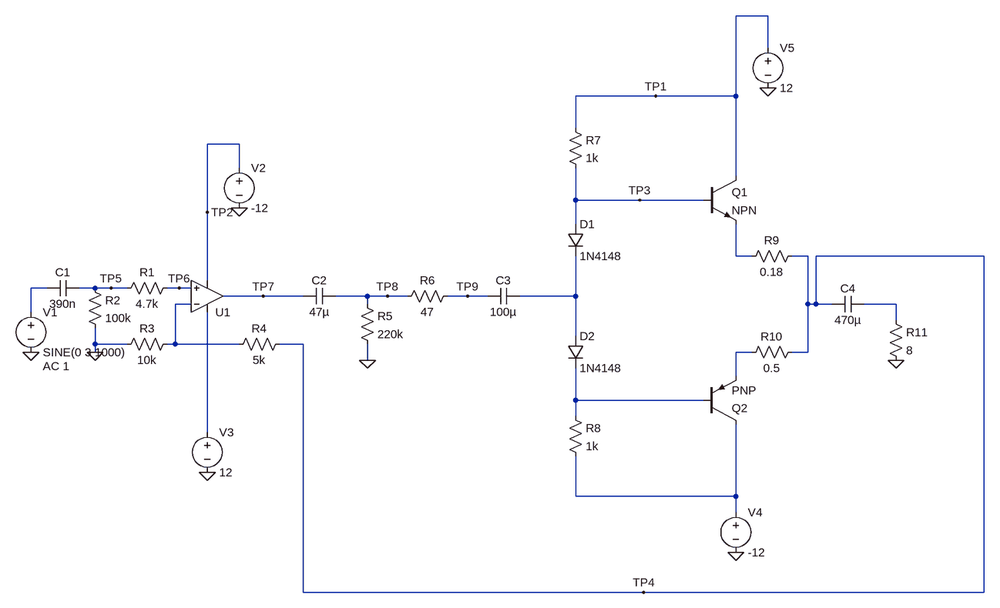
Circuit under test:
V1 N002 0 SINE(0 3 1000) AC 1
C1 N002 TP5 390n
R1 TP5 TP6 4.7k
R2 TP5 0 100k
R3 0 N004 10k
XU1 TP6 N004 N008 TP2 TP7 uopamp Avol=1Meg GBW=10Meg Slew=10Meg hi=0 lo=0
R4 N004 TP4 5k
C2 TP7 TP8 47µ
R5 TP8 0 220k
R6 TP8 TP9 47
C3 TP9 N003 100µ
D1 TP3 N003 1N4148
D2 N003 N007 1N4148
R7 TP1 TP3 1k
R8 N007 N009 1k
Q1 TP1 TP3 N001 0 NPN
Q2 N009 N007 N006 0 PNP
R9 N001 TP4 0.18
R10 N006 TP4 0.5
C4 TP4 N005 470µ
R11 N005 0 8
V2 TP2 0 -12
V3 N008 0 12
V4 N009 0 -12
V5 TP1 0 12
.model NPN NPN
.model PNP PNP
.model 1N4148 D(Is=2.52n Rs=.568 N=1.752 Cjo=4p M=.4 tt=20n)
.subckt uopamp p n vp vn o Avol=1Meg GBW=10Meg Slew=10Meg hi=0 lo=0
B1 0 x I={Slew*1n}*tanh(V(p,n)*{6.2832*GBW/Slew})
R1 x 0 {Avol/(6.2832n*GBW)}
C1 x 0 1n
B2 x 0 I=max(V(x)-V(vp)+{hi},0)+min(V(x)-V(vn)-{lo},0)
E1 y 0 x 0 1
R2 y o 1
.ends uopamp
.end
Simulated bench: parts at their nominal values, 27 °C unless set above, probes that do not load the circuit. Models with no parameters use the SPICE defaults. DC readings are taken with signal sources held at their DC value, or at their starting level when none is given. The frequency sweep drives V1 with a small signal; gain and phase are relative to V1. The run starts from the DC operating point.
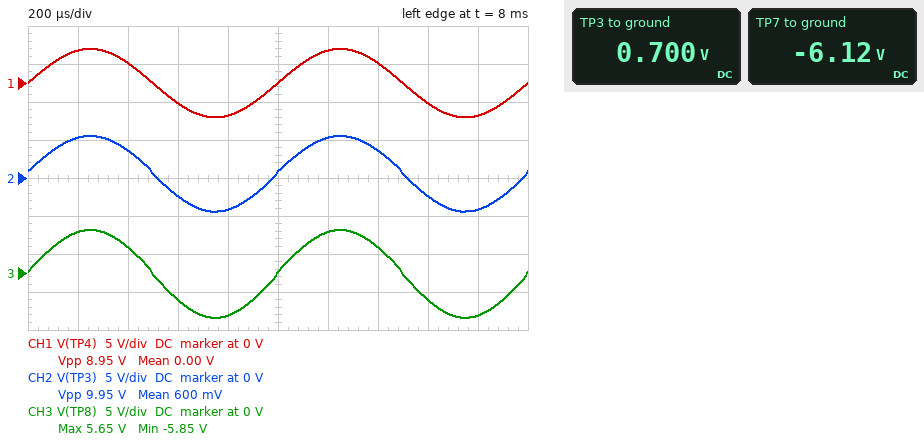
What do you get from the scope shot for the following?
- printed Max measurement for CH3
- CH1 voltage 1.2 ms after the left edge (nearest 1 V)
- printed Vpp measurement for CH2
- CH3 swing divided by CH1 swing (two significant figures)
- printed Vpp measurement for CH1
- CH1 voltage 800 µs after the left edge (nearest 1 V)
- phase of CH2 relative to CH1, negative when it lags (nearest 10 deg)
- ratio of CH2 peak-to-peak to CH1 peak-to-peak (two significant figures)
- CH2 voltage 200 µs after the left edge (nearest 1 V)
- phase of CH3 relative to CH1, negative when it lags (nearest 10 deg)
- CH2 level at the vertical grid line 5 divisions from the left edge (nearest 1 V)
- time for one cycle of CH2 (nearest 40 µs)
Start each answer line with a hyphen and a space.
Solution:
- 5.65 V
- 4 V
- 9.95 V
- 1.3
- 8.95 V
- -4 V
- 0 deg
- 1.1
- 5 V
- 0 deg
- 1 V
- 1.00 ms
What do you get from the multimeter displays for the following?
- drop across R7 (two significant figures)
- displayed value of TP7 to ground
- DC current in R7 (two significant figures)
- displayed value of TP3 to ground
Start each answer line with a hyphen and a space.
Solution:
- 11 V
- -6.12 V
- 11 mA
- 0.700 V
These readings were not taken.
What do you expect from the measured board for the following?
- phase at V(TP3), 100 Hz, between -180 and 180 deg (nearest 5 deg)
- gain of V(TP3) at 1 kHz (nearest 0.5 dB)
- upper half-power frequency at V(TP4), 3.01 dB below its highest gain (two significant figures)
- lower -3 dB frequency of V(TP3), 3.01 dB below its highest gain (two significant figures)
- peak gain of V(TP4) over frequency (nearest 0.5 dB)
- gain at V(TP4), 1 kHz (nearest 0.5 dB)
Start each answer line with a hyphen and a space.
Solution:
- 25 deg
- 32.5 dB
- 210 kHz
- 43 Hz
- 3.5 dB
- 3.5 dB
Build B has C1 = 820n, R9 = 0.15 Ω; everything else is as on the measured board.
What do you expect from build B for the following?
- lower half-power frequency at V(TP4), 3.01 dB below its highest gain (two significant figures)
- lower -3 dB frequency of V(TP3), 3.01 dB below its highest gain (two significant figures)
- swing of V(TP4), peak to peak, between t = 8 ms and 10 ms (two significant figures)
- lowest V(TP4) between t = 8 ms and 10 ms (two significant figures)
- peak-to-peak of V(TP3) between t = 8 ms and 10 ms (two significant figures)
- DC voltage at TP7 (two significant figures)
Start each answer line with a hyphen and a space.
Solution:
- 1.9 Hz
- 42 Hz
- 8.6 V
- -4.1 V
- 9.5 V
- -6.7 V
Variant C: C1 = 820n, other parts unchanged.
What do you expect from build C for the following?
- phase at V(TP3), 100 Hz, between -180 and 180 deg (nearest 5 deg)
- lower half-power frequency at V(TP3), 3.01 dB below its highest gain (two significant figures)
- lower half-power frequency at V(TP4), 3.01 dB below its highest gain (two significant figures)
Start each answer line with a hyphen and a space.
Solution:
- 25 deg
- 42 Hz
- 1.9 Hz
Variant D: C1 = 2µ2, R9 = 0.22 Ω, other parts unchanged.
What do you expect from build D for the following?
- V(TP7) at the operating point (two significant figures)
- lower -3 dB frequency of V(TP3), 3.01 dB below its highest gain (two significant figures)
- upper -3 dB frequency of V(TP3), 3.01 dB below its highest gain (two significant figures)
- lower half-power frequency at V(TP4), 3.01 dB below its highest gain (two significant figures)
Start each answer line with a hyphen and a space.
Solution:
- -5.4 V
- 42 Hz
- 210 kHz
- 720 mHz
